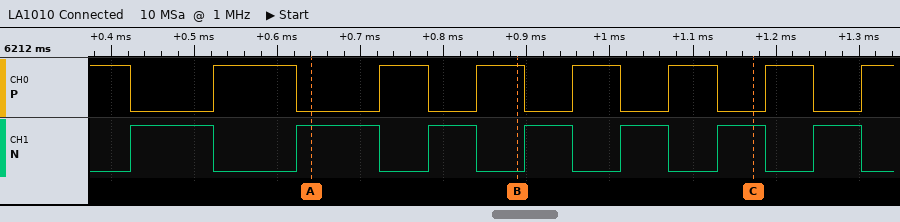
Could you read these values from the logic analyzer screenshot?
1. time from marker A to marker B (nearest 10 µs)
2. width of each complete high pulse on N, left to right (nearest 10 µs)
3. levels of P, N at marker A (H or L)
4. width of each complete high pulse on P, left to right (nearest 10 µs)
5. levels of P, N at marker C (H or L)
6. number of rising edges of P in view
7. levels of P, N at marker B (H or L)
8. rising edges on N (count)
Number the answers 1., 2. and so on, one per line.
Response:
1. 250 µs
2. 100 µs, 100 µs, 60 µs, 60 µs, 60 µs, 60 µs, 60 µs
3. P=L, N=H
4. 100 µs, 60 µs, 60 µs, 60 µs, 60 µs, 60 µs
5. P=L, N=H
6. 7
7. P=H, N=L
8. 7
